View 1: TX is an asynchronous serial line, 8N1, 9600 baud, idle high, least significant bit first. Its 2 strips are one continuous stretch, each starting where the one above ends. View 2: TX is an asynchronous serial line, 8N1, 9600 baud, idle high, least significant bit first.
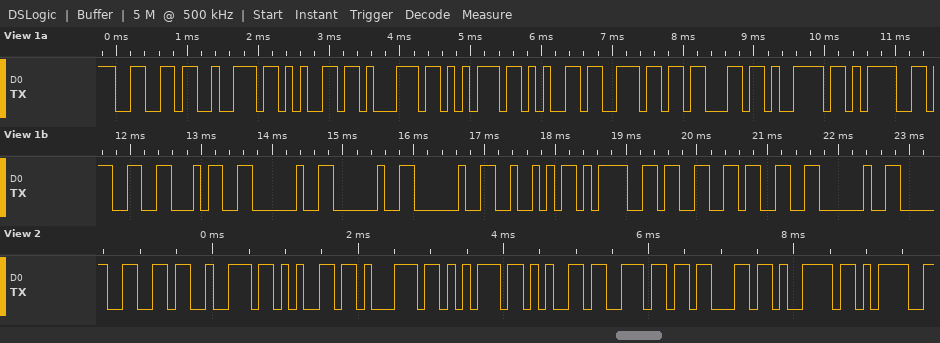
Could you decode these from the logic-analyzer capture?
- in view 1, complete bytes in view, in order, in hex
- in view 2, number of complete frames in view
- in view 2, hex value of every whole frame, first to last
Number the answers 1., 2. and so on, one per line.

1. 0x66 0x72 0x65 0x71 0x75 0x65 0x6E 0x63 0x79 0x3D 0x33 0x34 0x20 0x20 0x20 0x52 0x3D 0x33 0x33 0x20
2. 10
3. 66 72 65 71 75 65 6E 63 79 3D
